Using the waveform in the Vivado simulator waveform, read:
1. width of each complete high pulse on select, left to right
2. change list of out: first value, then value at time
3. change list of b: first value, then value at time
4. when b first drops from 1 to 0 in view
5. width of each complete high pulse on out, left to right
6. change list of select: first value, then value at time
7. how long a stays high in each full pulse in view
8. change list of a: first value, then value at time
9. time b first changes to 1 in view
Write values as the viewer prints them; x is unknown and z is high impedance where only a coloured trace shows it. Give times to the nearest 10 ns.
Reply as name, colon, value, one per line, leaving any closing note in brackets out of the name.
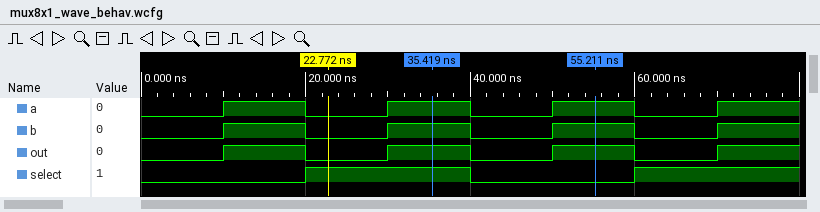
width of each complete high pulse on select, left to right: 20 ns
change list of out: first value, then value at time: 0, 1 at 10 ns, 0 at 20 ns, 1 at 30 ns, 0 at 40 ns, 1 at 50 ns, 0 at 60 ns, 1 at 70 ns
change list of b: first value, then value at time: 0, 1 at 10 ns, 0 at 20 ns, 1 at 30 ns, 0 at 40 ns, 1 at 50 ns, 0 at 60 ns, 1 at 70 ns
when b first drops from 1 to 0 in view: 20 ns
width of each complete high pulse on out, left to right: 10 ns, 10 ns, 10 ns
change list of select: first value, then value at time: 0, 1 at 20 ns, 0 at 40 ns, 1 at 60 ns
how long a stays high in each full pulse in view: 10 ns, 10 ns, 10 ns
change list of a: first value, then value at time: 0, 1 at 10 ns, 0 at 20 ns, 1 at 30 ns, 0 at 40 ns, 1 at 50 ns, 0 at 60 ns, 1 at 70 ns
time b first changes to 1 in view: 10 ns
